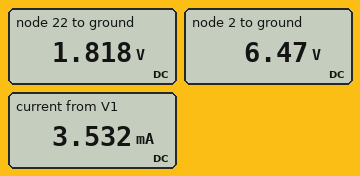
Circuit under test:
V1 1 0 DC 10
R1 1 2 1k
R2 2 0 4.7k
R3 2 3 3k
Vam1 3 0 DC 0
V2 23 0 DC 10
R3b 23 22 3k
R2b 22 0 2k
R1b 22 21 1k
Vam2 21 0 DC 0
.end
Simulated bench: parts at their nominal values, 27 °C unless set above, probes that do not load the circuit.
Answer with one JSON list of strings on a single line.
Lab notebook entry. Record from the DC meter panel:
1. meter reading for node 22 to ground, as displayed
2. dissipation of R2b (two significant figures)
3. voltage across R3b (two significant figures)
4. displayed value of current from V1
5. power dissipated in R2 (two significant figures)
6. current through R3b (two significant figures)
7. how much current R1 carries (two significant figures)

["1.818 V", "1.7 mW", "8.2 V", "3.532 mA", "8.9 mW", "2.7 mA", "3.5 mA"]
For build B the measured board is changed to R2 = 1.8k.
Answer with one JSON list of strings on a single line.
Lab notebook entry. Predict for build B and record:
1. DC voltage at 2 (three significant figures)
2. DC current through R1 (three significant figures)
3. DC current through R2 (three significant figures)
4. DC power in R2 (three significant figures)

["5.29 V", "4.71 mA", "2.94 mA", "15.6 mW"]
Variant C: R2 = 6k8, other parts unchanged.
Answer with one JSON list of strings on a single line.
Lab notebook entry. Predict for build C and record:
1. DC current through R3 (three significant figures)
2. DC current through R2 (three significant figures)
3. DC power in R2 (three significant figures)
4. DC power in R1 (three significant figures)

["2.25 mA", "993 µA", "6.71 mW", "10.5 mW"]
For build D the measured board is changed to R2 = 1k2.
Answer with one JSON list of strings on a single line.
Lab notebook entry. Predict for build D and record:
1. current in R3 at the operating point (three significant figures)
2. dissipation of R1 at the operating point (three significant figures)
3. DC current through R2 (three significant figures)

["1.54 mA", "29.0 mW", "3.85 mA"]
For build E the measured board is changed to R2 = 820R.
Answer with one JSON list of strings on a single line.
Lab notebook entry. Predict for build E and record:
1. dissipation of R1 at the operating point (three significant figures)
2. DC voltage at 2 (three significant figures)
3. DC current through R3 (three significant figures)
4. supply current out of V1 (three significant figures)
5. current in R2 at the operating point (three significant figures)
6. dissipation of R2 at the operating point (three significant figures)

["37.0 mW", "3.92 V", "1.31 mA", "6.08 mA", "4.78 mA", "18.7 mW"]
